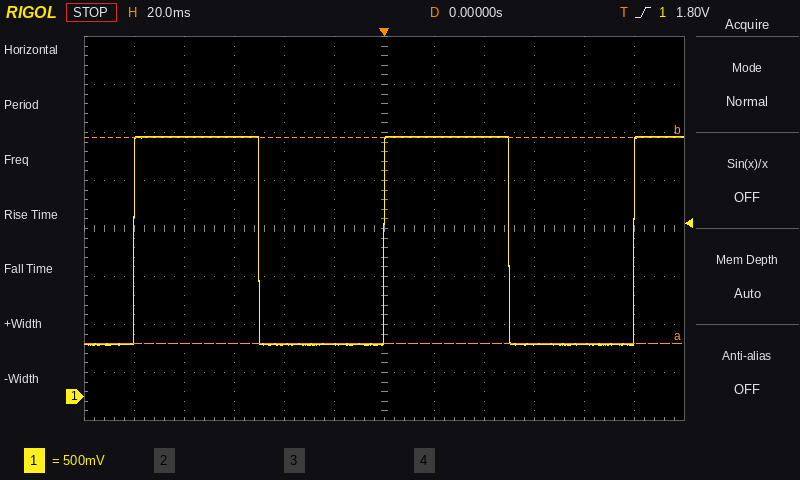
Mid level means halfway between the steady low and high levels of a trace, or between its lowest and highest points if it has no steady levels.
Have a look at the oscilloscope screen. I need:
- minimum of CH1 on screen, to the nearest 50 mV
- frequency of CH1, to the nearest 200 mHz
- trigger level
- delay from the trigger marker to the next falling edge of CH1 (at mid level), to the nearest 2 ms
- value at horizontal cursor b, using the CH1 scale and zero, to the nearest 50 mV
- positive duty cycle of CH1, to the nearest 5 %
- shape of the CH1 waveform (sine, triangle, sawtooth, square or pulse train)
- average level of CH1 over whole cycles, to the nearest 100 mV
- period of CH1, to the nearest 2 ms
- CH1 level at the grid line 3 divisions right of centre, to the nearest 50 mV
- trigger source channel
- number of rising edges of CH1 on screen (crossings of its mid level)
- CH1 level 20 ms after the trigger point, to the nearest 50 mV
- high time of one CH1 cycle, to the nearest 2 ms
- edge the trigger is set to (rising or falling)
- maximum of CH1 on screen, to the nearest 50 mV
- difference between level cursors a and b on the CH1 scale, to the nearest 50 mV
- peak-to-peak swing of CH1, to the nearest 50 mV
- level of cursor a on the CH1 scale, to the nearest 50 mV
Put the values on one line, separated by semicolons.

550 mV; 10.0 Hz; 1.80 V; 50 ms; 2.70 V; 50 %; square; 1.6 V; 100 ms; 550 mV; CH1; 3; 2.70 V; 50 ms; rising; 2.70 V; 2.15 V; 2.15 V; 550 mV
